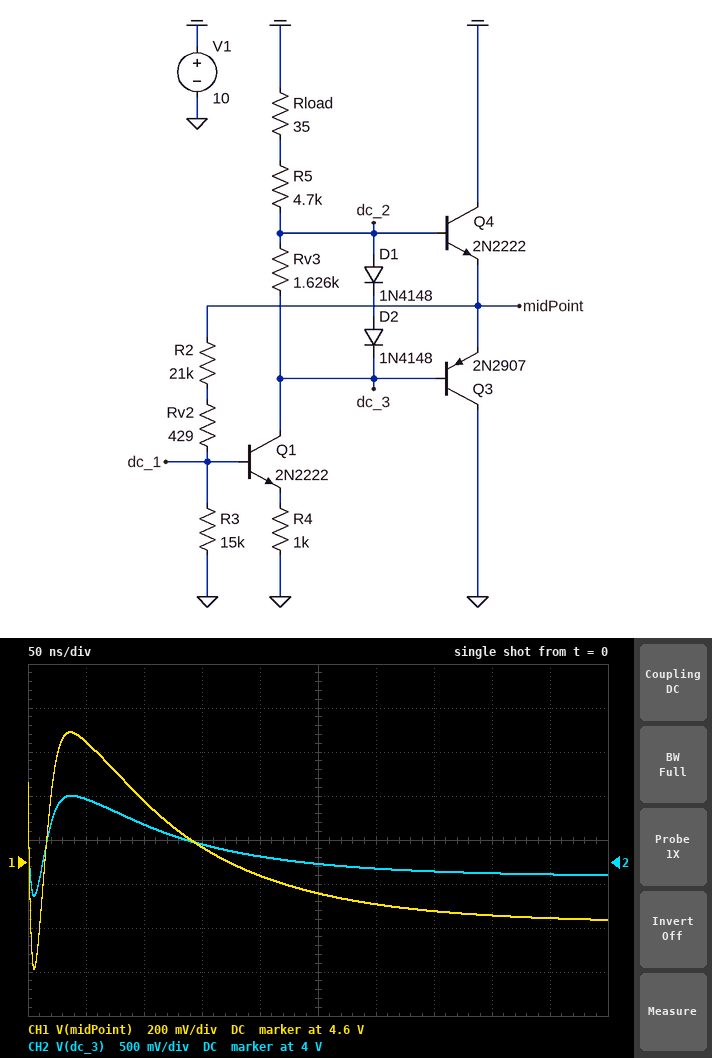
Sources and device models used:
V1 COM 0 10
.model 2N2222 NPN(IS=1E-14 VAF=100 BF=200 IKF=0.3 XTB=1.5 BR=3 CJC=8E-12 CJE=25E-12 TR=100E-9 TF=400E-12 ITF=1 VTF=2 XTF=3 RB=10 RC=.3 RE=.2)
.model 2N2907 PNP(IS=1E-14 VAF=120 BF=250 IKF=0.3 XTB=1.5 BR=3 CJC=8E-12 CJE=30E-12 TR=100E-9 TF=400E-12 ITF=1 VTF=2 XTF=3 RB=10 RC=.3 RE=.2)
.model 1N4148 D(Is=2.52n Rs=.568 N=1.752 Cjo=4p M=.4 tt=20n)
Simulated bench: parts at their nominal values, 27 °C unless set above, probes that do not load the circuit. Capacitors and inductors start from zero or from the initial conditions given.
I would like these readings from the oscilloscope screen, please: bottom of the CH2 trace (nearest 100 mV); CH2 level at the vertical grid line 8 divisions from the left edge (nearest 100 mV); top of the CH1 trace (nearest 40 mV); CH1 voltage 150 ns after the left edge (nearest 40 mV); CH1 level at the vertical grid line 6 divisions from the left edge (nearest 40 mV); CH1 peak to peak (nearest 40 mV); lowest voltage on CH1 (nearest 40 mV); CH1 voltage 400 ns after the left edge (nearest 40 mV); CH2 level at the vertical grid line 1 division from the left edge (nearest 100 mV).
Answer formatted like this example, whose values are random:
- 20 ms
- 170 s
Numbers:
- 3.6 V
- 3.9 V
- 5.20 V
- 4.68 V
- 4.40 V
- 1.08 V
- 4.12 V
- 4.36 V
- 4.7 V
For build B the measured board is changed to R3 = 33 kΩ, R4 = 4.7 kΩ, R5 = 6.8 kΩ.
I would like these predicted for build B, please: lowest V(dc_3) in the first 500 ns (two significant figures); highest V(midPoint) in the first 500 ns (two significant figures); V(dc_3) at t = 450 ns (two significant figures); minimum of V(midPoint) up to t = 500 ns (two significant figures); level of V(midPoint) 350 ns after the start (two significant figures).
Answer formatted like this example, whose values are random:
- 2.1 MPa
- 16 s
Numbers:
- 4.3 V
- 5.8 V
- 5.3 V
- 4.8 V
- 5.6 V
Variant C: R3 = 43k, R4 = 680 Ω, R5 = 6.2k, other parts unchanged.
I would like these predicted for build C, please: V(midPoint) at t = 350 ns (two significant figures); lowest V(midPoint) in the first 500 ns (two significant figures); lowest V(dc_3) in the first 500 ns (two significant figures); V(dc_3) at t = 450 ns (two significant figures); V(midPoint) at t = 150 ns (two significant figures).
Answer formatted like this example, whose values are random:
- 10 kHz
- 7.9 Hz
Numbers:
- 2.5 V
- 2.4 V
- 1.8 V
- 1.9 V
- 3.2 V
